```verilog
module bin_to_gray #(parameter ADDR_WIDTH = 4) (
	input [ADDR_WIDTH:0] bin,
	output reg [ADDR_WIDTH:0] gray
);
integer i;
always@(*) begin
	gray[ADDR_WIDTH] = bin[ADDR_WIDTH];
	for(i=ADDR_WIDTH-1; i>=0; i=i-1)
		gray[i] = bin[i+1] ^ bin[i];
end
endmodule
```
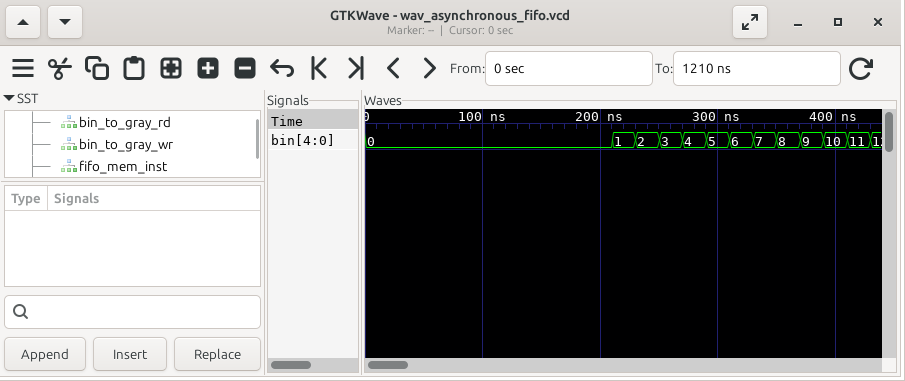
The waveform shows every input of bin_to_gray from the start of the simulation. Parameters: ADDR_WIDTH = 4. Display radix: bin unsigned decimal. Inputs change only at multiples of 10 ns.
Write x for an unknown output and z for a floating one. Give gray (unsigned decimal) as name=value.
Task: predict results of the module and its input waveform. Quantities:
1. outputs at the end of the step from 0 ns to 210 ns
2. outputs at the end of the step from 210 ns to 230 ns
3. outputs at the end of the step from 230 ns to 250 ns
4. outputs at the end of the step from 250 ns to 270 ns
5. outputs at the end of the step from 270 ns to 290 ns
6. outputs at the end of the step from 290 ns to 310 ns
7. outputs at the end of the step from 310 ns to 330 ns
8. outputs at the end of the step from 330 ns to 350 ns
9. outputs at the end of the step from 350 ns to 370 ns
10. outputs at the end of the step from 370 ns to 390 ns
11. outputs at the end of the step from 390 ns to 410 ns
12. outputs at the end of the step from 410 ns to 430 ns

gray=0
gray=1
gray=3
gray=2
gray=6
gray=7
gray=5
gray=4
gray=12
gray=13
gray=15
gray=14
